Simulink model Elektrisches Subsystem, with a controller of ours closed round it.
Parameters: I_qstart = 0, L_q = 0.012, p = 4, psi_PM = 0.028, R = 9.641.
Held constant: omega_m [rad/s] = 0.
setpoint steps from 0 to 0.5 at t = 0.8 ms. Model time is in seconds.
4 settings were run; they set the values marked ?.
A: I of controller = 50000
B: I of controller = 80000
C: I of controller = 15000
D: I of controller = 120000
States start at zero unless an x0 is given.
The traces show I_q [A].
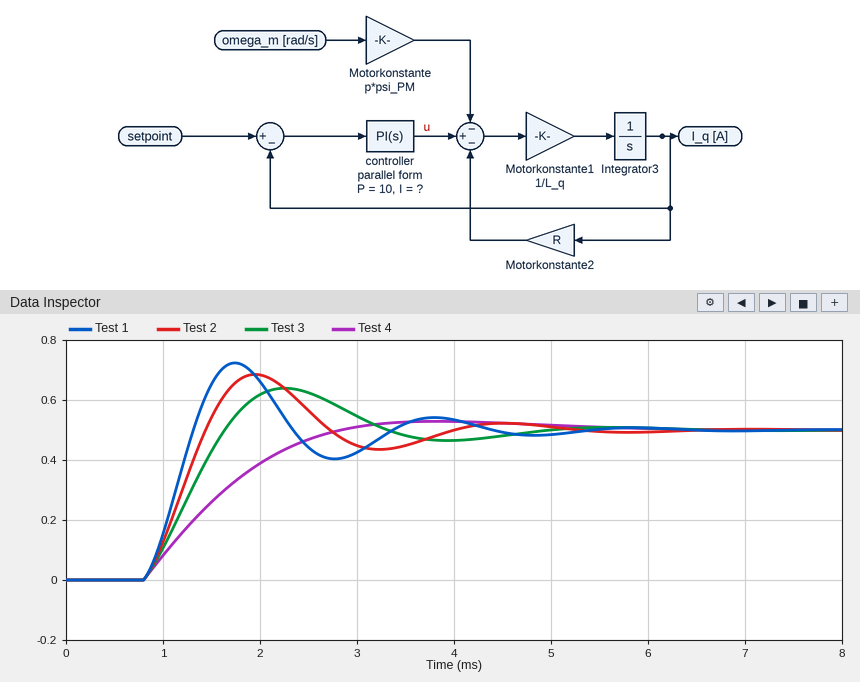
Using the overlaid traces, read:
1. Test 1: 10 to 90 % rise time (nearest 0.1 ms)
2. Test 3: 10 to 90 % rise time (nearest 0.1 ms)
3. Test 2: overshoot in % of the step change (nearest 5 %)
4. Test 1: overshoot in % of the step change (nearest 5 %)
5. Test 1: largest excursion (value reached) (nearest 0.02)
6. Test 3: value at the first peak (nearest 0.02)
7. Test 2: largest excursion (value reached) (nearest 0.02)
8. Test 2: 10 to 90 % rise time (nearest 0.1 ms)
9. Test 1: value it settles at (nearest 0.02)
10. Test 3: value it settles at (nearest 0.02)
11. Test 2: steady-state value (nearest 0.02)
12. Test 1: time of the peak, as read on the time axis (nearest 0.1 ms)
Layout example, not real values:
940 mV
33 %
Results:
0.4 ms
0.6 ms
35 %
45 %
0.72
0.64
0.68
0.5 ms
0.50
0.50
0.50
1.7 ms
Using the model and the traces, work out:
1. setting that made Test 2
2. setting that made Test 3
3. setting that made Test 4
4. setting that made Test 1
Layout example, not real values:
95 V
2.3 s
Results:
B
A
C
D
